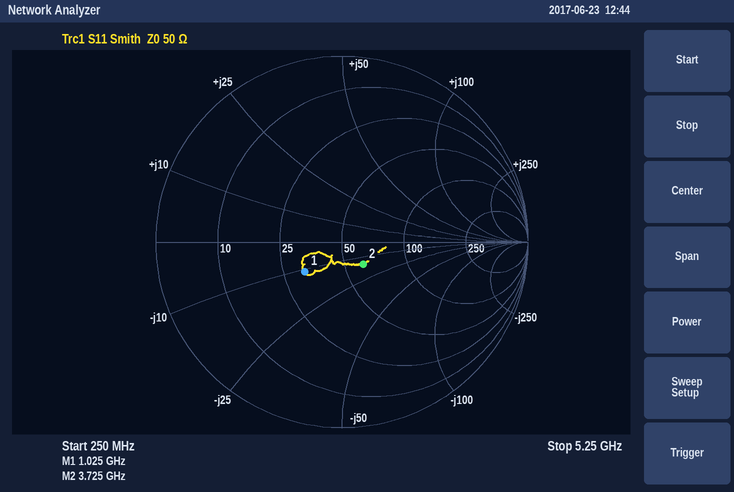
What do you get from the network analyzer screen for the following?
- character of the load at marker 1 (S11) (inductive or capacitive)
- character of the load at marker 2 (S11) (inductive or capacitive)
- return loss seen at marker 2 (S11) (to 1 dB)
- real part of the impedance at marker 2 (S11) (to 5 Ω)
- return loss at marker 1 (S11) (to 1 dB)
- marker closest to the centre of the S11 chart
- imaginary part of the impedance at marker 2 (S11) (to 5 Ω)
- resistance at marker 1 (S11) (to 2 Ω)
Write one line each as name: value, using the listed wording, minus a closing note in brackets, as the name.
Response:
character of the load at marker 1 (S11): capacitive
character of the load at marker 2 (S11): capacitive
return loss seen at marker 2 (S11): 16 dB
real part of the impedance at marker 2 (S11): 60 Ω
return loss at marker 1 (S11): 12 dB
marker closest to the centre of the S11 chart: marker 2
imaginary part of the impedance at marker 2 (S11): -15 Ω
resistance at marker 1 (S11): 32 Ω
